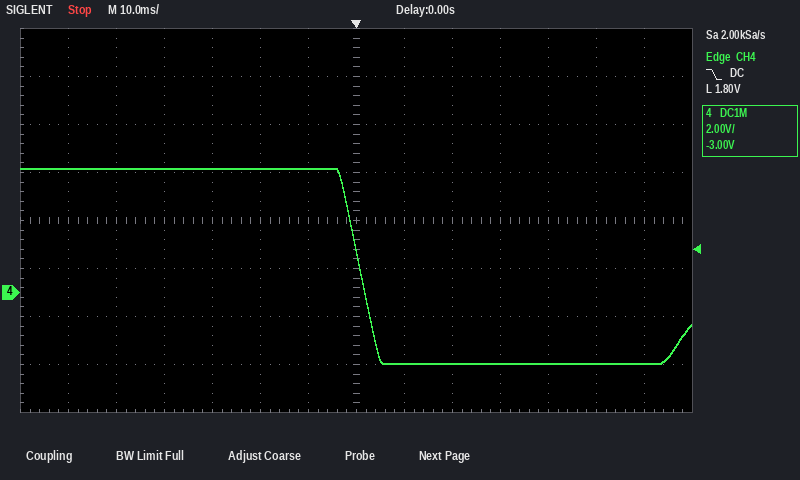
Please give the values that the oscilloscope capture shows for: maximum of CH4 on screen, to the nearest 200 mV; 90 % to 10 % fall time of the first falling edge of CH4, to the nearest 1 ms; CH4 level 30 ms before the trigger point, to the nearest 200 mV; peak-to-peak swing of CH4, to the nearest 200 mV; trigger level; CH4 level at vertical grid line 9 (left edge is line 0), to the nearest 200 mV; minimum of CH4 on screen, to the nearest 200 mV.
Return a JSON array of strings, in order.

["5.2 V", "7 ms", "5.2 V", "8.2 V", "1.80 V", "-3.0 V", "-3.0 V"]
